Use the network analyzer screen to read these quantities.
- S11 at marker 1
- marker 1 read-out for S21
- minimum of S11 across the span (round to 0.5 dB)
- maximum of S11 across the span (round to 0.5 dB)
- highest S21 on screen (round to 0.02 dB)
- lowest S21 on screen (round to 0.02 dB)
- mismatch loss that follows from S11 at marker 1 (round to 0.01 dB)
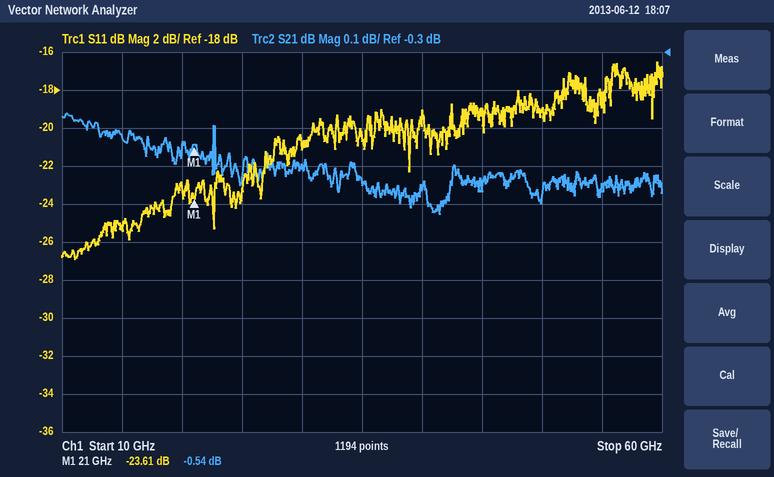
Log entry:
-23.61 dB
-0.54 dB
-27.0 dB
-16.5 dB
-0.46 dB
-0.72 dB
0.02 dB
